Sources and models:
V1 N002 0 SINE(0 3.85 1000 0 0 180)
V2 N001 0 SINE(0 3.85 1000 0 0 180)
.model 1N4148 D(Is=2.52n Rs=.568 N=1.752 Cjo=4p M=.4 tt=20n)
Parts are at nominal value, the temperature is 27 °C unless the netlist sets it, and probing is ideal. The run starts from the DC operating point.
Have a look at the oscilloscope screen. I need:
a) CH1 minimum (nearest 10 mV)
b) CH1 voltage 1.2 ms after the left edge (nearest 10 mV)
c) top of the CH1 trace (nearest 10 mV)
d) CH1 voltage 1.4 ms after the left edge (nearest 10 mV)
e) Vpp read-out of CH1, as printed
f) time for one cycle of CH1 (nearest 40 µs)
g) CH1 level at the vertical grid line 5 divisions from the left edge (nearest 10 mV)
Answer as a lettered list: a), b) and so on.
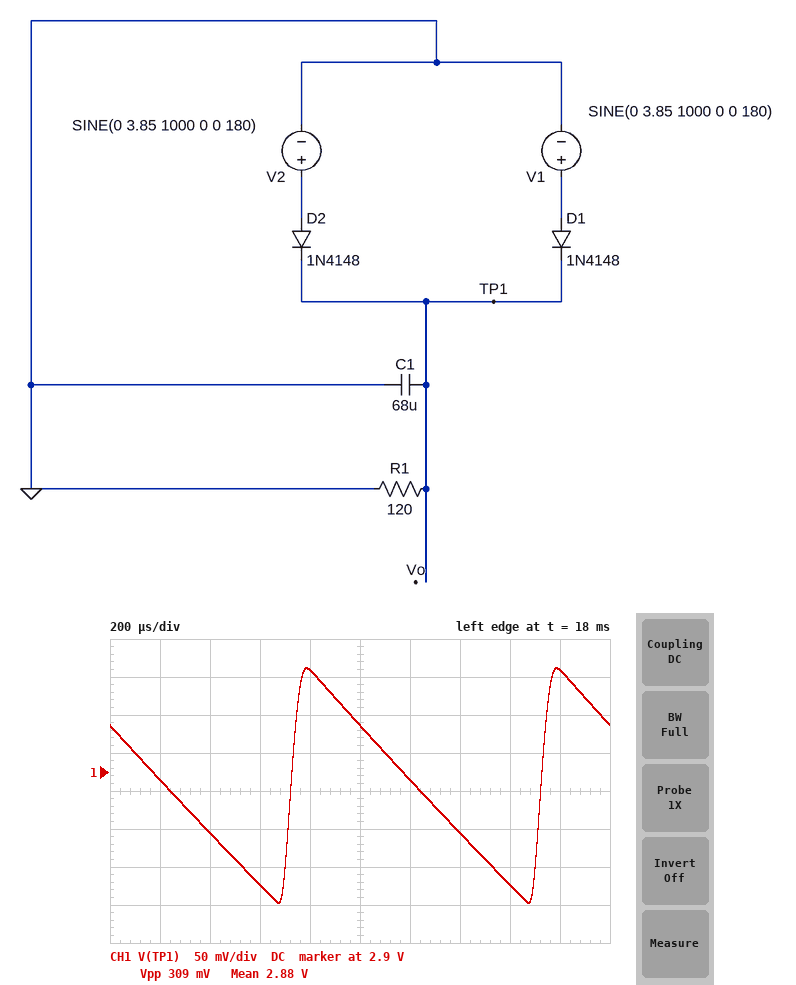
a) 2.73 V
b) 2.89 V
c) 3.04 V
d) 2.82 V
e) 309 mV
f) 1.00 ms
g) 2.96 V
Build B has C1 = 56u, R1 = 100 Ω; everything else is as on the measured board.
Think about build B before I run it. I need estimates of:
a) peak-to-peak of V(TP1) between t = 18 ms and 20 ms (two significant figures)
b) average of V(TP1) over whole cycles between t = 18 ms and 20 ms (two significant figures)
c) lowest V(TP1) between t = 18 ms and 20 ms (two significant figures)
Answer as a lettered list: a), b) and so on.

a) 440 mV
b) 2.8 V
c) 2.6 V
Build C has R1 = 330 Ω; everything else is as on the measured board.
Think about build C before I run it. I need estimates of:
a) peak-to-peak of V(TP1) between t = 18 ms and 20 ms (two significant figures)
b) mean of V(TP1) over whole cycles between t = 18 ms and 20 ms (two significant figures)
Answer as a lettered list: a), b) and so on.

a) 120 mV
b) 3.0 V
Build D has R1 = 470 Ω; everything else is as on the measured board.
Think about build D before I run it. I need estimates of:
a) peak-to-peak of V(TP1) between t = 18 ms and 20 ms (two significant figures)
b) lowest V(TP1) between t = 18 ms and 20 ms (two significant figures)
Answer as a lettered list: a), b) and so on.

a) 85 mV
b) 3.0 V
